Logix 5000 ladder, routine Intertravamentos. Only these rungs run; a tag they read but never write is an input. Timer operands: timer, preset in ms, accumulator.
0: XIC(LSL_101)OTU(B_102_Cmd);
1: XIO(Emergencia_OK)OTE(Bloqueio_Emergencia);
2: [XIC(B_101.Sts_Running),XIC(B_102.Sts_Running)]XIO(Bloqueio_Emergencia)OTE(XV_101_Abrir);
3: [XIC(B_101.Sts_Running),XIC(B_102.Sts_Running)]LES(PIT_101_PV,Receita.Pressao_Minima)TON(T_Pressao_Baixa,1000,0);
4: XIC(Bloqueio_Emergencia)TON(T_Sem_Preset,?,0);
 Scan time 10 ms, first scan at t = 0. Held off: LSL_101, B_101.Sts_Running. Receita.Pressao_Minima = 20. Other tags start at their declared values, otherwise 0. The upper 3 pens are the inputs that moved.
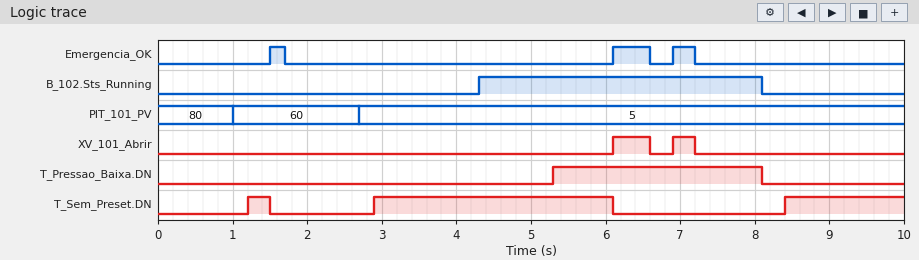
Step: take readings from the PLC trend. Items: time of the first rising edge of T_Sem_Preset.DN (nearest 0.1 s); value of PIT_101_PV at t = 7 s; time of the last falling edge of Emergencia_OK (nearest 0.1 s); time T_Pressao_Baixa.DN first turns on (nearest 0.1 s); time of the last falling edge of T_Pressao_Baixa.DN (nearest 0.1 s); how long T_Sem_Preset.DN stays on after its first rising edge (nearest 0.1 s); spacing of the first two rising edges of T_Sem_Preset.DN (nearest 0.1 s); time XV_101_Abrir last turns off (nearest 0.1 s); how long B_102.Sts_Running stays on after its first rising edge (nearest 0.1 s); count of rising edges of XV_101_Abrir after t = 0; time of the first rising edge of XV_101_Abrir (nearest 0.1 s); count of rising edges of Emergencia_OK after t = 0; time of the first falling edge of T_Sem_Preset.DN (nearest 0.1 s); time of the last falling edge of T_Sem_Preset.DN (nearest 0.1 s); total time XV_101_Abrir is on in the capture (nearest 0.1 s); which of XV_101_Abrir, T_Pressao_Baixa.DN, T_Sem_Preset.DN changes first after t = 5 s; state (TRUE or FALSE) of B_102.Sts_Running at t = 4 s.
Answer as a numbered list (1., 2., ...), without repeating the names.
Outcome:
1. 1.2 s
2. 5
3. 7.2 s
4. 5.3 s
5. 8.1 s
6. 0.3 s
7. 1.7 s
8. 7.2 s
9. 3.8 s
10. 2
11. 6.1 s
12. 3
13. 1.5 s
14. 6.1 s
15. 0.8 s
16. T_Pressao_Baixa.DN
17. FALSE
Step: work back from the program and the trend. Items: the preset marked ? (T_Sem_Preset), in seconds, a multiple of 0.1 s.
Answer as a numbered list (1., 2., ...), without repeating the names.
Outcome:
1. 1.2 s
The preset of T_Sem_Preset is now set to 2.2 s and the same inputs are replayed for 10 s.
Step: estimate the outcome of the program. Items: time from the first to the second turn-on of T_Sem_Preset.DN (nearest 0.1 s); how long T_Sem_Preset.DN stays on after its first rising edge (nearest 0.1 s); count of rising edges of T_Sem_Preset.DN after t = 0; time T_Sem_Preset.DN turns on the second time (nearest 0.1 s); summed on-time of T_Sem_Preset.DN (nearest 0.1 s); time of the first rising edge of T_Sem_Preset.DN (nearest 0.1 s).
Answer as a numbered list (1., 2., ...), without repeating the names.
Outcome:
1. 5.5 s
2. 2.2 s
3. 2
4. 9.4 s
5. 2.8 s
6. 3.9 s
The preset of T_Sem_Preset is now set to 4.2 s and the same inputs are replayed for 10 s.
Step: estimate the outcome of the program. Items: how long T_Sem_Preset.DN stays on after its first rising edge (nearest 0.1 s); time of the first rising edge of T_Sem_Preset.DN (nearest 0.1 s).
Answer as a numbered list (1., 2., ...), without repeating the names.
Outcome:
1. 0.2 s
2. 5.9 s
